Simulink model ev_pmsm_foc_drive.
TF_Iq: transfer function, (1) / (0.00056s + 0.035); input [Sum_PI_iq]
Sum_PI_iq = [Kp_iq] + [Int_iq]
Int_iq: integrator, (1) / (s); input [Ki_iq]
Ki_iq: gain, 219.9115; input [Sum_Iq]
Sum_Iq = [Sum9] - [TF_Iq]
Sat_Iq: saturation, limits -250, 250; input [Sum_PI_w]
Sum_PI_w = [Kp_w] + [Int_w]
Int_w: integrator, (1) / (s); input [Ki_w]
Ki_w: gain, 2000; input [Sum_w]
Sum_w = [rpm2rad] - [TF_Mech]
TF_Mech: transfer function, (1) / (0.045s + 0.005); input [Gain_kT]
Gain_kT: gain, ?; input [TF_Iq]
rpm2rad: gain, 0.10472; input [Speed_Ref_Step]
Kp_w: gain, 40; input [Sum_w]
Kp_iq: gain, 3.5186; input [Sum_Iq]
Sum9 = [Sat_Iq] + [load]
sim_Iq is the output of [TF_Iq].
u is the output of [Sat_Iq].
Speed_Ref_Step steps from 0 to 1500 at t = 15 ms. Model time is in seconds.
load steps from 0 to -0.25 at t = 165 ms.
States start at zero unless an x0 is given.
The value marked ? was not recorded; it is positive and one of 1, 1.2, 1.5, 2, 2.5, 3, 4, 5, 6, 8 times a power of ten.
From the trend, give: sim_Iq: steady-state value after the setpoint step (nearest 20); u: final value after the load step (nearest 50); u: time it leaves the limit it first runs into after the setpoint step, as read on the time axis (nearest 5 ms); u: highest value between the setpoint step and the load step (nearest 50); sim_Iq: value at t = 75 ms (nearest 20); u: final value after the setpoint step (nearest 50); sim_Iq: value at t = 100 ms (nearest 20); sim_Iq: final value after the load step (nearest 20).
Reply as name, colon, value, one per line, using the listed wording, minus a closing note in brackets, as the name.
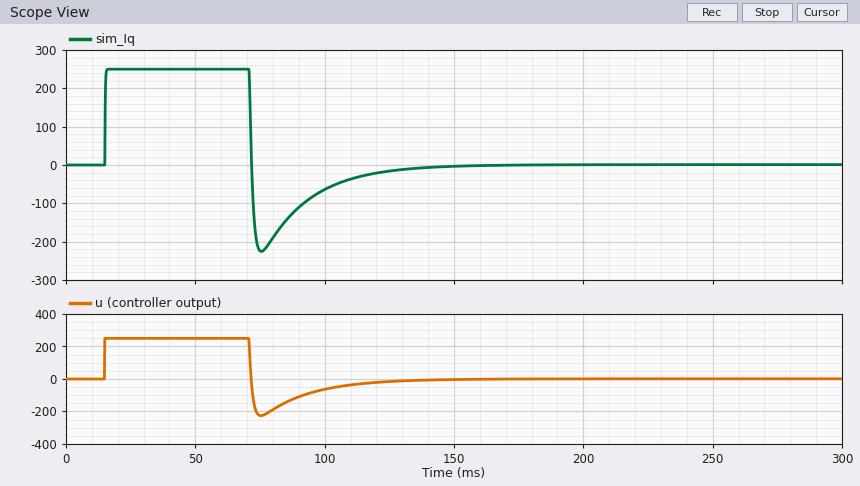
sim_Iq: steady-state value after the setpoint step: 0
u: final value after the load step: 0
u: time it leaves the limit it first runs into after the setpoint step, as read on the time axis: 70 ms
u: highest value between the setpoint step and the load step: 250
sim_Iq: value at t = 75 ms: -220
u: final value after the setpoint step: 0
sim_Iq: value at t = 100 ms: -60
sim_Iq: final value after the load step: 0
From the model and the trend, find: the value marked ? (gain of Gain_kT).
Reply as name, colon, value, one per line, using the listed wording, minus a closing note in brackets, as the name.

the value marked ?: 0.8
